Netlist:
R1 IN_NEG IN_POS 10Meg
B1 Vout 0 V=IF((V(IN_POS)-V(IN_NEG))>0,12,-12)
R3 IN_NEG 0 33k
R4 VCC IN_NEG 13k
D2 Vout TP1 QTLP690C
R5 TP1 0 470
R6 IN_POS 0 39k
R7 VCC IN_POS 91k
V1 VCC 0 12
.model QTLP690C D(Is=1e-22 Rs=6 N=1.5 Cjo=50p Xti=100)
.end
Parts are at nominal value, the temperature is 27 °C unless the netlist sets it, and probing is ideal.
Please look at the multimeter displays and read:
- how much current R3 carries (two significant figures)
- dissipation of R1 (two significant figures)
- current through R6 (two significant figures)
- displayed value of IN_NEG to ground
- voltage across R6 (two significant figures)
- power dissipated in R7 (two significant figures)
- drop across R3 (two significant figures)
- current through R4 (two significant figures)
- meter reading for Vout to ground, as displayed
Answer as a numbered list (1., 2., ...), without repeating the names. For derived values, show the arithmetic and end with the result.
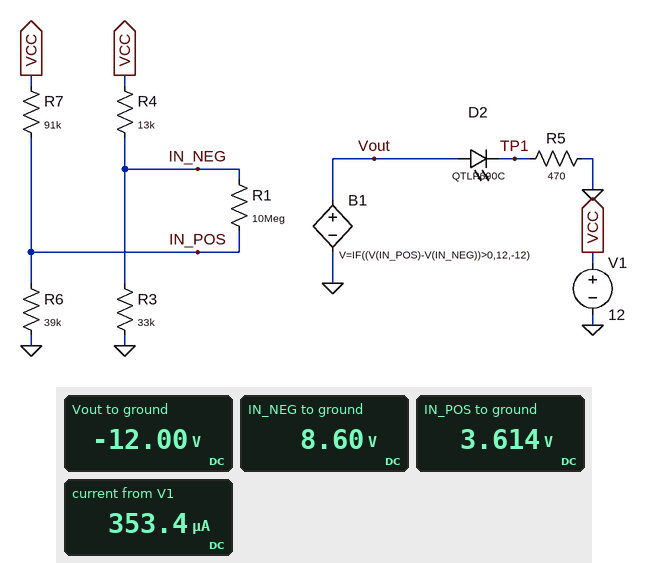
1. (8.6 V) / 33 kΩ = 260 µA
2. (8.6 V - 3.614 V)^2 / 10 MΩ = 2.5 µW
3. (3.614 V) / 39 kΩ = 93 µA
4. 8.60 V
5. 3.614 V = 3.6 V
6. (12 V - 3.614 V)^2 / 91 kΩ = 770 µW
7. 8.6 V = 8.6 V
8. (12 V - 8.6 V) / 13 kΩ = 260 µA
9. -12.00 V
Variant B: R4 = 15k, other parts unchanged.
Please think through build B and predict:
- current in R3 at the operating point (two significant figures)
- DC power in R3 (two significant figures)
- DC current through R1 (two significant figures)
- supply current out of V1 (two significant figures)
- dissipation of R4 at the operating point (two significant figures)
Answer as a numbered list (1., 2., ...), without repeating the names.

1. 250 µA
2. 2.1 mW
3. 460 nA
4. 340 µA
5. 940 µW
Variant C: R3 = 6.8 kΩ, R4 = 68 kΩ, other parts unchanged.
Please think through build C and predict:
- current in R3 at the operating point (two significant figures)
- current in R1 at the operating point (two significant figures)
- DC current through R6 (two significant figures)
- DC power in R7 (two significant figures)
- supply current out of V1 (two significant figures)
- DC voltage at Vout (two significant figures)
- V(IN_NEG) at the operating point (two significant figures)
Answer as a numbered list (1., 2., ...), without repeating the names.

1. 160 µA
2. 250 nA
3. 92 µA
4. 780 µW
5. 250 µA
6. 12 V
7. 1.1 V
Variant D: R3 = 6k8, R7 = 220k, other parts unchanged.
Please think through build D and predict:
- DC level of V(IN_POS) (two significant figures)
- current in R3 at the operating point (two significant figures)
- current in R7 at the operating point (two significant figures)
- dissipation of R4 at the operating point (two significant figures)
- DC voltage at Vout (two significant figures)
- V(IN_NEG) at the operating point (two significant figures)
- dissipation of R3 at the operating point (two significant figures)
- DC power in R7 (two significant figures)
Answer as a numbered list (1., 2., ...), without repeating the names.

1. 1.8 V
2. 610 µA
3. 46 µA
4. 4.8 mW
5. -12 V
6. 4.1 V
7. 2.5 mW
8. 470 µW
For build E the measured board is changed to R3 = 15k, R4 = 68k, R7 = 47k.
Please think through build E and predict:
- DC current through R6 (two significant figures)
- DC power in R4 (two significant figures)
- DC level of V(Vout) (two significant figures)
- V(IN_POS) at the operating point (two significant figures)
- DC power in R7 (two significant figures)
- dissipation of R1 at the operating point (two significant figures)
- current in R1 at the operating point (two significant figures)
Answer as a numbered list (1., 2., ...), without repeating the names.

1. 140 µA
2. 1.4 mW
3. 12 V
4. 5.4 V
5. 920 µW
6. 1.1 µW
7. 330 nA
